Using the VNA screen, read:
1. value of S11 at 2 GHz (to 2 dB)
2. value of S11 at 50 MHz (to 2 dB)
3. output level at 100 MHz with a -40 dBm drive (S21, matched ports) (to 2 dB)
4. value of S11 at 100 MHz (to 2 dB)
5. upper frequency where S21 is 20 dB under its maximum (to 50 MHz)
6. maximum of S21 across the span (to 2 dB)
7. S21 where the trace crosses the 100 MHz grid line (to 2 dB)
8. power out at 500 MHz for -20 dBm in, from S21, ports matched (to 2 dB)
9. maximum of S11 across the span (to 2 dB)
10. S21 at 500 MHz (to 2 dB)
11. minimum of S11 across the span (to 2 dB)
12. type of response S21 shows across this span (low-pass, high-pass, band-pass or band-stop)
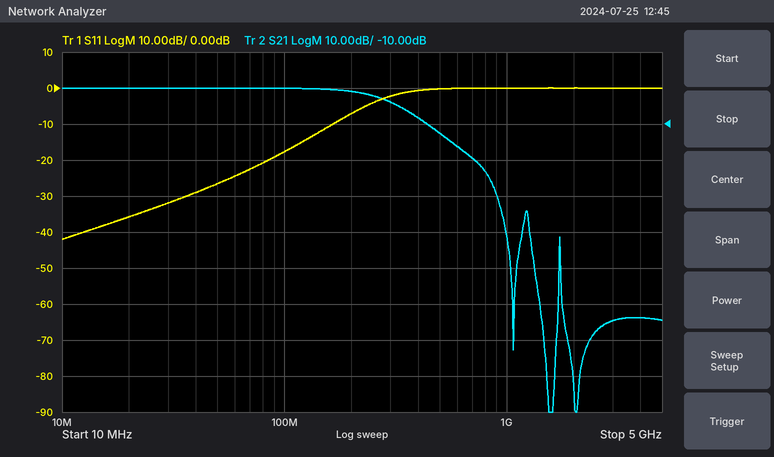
0 dB
-26 dB
-40 dBm
-18 dB
700 MHz
0 dB
0 dB
-32 dBm
0 dB
-12 dB
-42 dB
low-pass
